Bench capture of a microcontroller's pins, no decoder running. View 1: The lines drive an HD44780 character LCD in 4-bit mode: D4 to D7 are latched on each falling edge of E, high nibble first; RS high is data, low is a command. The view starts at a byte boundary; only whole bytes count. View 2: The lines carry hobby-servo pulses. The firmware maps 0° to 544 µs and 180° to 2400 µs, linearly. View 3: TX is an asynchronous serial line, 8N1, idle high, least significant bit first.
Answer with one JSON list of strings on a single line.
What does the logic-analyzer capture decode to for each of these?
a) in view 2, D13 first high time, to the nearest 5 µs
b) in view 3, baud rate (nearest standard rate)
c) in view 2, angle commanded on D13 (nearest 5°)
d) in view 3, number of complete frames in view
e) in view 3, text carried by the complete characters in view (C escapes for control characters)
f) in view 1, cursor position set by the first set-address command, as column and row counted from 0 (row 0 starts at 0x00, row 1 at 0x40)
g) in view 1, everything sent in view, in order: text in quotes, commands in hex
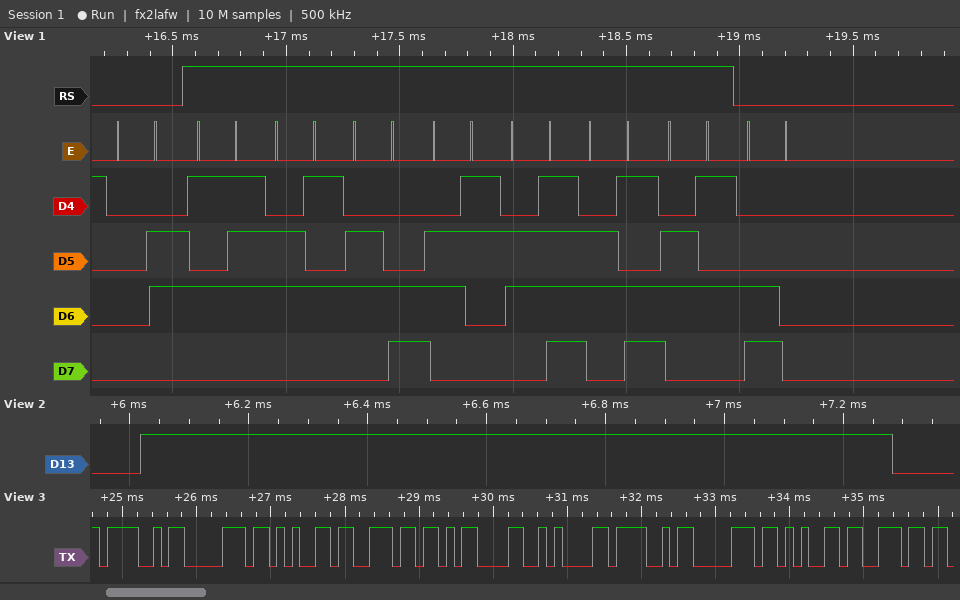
["1265 µs", "9600 baud", "70°", "10", "\"Open\\r\\nOpen\"", "column 0, row 1", "0x06 \"Welcome\" 0xC0"]
